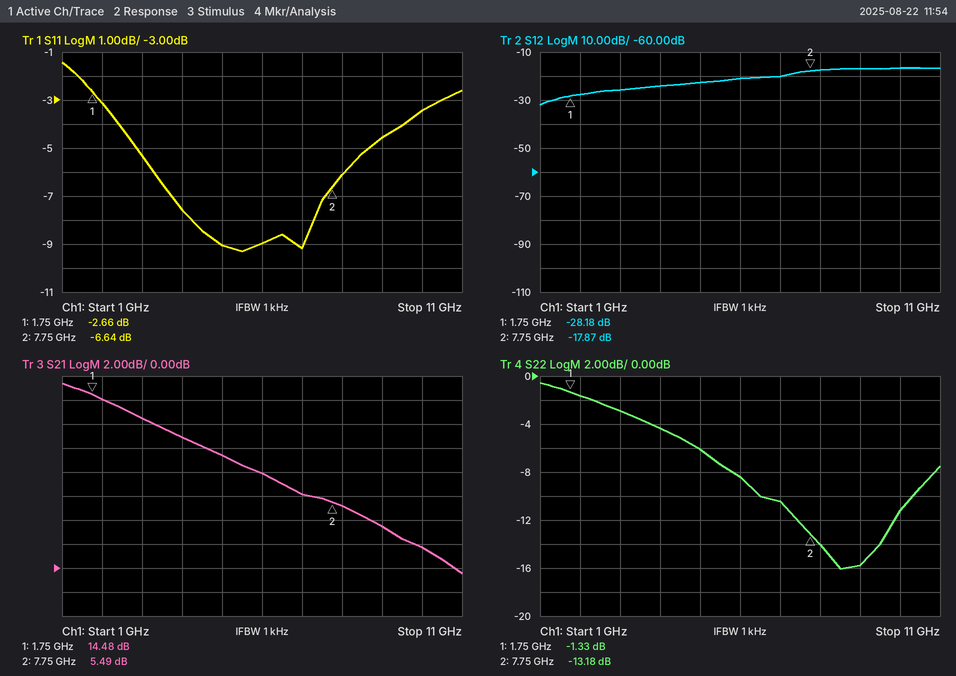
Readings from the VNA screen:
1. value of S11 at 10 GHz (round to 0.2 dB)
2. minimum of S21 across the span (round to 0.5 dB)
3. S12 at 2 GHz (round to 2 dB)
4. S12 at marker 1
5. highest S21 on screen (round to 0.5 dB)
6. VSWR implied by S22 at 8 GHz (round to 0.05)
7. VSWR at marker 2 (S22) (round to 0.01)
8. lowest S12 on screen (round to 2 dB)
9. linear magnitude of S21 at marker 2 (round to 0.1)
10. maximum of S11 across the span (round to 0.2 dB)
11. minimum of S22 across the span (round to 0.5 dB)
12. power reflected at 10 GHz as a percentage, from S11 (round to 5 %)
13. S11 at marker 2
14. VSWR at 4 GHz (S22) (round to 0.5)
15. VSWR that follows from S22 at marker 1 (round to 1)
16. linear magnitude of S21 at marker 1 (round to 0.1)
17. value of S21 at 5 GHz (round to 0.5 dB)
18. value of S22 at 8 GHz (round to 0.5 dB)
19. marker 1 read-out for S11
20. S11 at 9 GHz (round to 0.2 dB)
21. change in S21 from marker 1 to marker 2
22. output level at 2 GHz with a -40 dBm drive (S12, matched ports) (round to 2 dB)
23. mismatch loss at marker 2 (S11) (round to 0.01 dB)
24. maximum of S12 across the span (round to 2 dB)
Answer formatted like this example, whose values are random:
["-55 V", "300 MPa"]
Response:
["-3.4 dB", "-0.5 dB", "-28 dB", "-28.18 dB", "15.5 dB", "1.50", "1.56", "-32 dB", "1.9", "-1.4 dB", "-16.0 dB", "45 %", "-6.64 dB", "4.0", "13", "5.3", "9.5 dB", "-14.0 dB", "-2.66 dB", "-4.6 dB", "-8.99 dB", "-68 dBm", "1.06 dB", "-16 dB"]
